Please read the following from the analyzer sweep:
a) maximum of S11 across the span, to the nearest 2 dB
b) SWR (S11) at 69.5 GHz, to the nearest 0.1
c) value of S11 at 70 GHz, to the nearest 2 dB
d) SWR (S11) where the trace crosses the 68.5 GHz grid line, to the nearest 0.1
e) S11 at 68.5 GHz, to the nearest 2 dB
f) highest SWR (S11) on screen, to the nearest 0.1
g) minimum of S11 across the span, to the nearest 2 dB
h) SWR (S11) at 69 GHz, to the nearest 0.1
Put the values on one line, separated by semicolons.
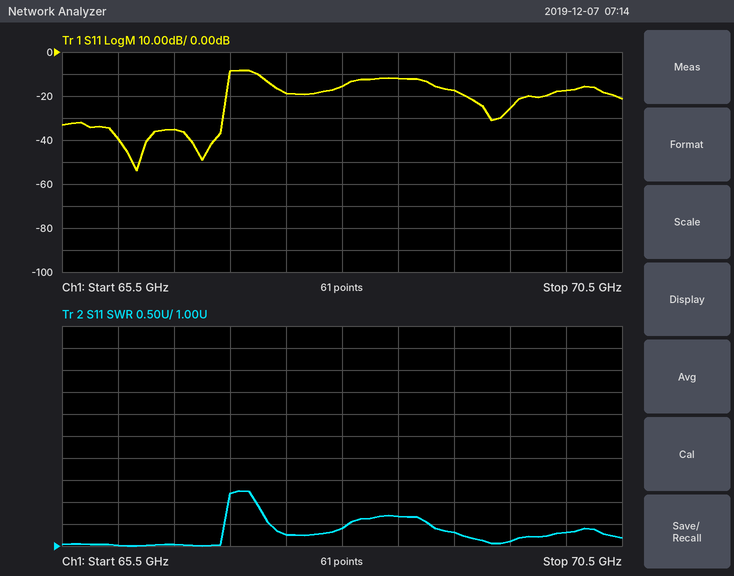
-8 dB; 1.1; -18 dB; 1.7; -12 dB; 2.3; -54 dB; 1.3
